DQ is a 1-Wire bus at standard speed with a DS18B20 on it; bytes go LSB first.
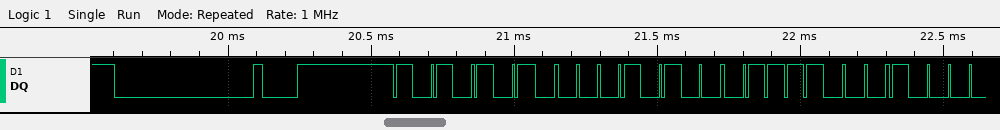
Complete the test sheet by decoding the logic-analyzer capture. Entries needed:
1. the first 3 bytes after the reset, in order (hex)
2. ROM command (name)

55 28 1E
Match ROM
